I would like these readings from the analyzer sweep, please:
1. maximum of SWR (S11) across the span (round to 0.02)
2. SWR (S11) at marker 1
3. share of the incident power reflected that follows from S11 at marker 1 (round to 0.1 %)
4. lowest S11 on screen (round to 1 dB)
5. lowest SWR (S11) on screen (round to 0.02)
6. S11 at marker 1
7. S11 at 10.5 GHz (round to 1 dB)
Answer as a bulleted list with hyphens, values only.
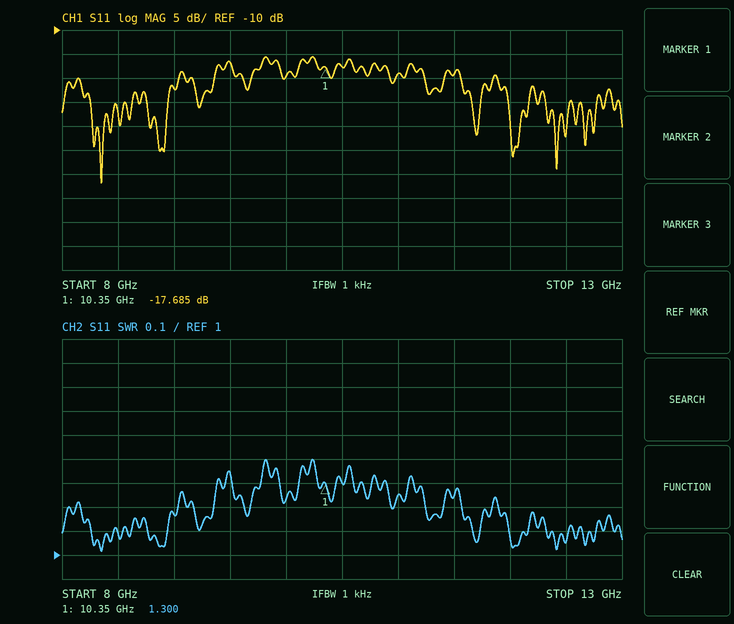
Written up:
- 1.40
- 1.300
- 1.7 %
- -42 dB
- 1.02
- -17.685 dB
- -18 dB
